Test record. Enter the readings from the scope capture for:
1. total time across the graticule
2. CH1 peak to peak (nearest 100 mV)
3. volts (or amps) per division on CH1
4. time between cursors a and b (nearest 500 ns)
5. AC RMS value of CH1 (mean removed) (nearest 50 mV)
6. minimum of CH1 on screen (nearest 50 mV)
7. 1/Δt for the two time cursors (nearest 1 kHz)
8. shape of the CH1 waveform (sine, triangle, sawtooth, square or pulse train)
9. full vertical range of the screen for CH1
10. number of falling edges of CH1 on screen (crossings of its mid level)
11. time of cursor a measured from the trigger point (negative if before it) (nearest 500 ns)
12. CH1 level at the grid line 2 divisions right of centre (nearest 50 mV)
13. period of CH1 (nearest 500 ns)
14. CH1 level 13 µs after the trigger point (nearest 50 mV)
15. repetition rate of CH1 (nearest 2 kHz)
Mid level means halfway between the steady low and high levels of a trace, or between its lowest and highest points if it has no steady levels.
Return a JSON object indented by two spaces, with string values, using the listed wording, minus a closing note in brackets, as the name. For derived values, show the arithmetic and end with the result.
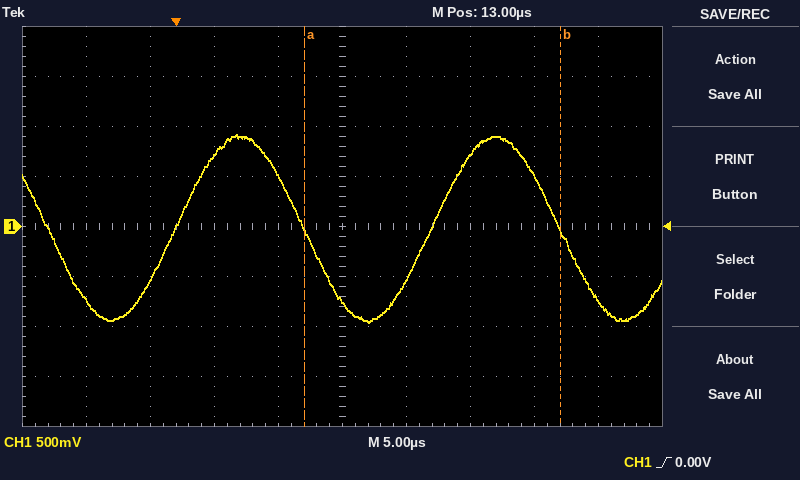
{
  "total time across the graticule": "50 µs",
  "CH1 peak to peak": "1.90 V",
  "volts (or amps) per division on CH1": "500 mV",
  "time between cursors a and b": "20.0 µs",
  "AC RMS value of CH1 (mean removed)": "1.90 V / (2√2) ≈ 672 mV, so 650 mV to the nearest 50 mV",
  "minimum of CH1 on screen": "-950 mV",
  "1/Δt for the two time cursors": "1 / 20.0 µs ≈ 50 kHz",
  "shape of the CH1 waveform": "sine",
  "full vertical range of the screen for CH1": "4 V",
  "number of falling edges of CH1 on screen": "3",
  "time of cursor a measured from the trigger point (negative if before it)": "+10.0 µs",
  "CH1 level at the grid line 2 divisions right of centre": "700 mV",
  "period of CH1": "20.0 µs",
  "CH1 level 13 µs after the trigger point": "-750 mV",
  "repetition rate of CH1": "1 / 20.0 µs ≈ 50 kHz"
}
